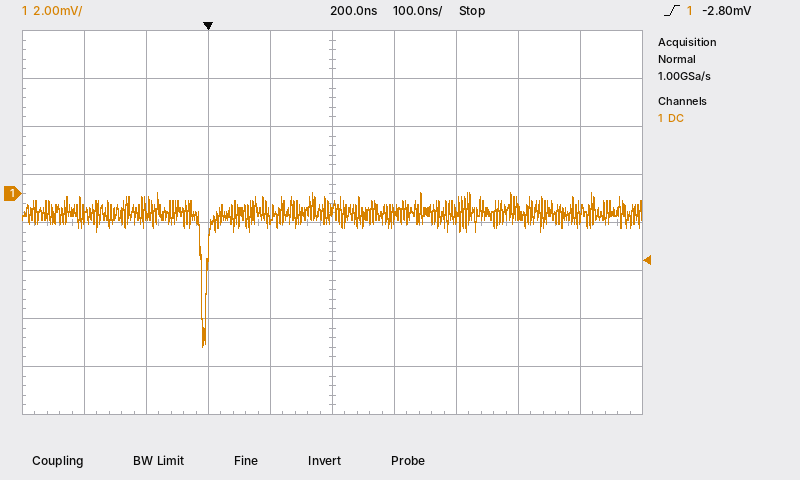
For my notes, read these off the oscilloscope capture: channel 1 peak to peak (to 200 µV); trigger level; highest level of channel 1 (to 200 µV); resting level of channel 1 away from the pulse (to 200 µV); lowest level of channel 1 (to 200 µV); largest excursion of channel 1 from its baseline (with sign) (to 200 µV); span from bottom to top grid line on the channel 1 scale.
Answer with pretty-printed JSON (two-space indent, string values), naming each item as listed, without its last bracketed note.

{
  "channel 1 peak to peak": "6.4 mV",
  "trigger level": "-2.80 mV",
  "highest level of channel 1": "0.0 mV",
  "resting level of channel 1 away from the pulse": "-800 µV",
  "lowest level of channel 1": "-6.4 mV",
  "largest excursion of channel 1 from its baseline (with sign)": "-5.6 mV",
  "span from bottom to top grid line on the channel 1 scale": "16 mV"
}
